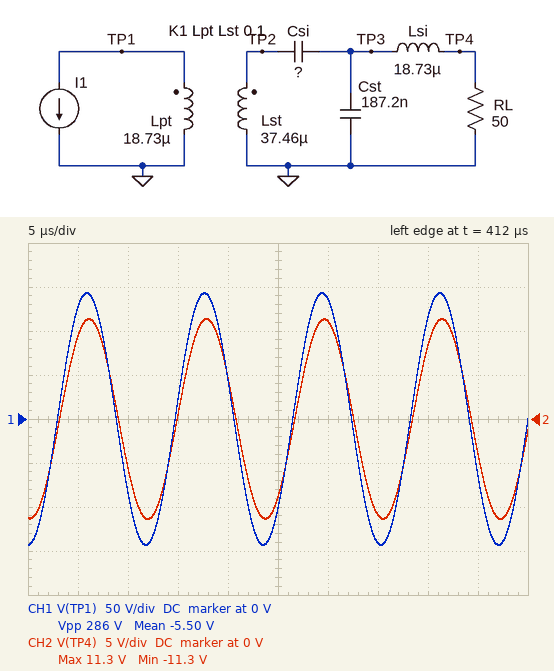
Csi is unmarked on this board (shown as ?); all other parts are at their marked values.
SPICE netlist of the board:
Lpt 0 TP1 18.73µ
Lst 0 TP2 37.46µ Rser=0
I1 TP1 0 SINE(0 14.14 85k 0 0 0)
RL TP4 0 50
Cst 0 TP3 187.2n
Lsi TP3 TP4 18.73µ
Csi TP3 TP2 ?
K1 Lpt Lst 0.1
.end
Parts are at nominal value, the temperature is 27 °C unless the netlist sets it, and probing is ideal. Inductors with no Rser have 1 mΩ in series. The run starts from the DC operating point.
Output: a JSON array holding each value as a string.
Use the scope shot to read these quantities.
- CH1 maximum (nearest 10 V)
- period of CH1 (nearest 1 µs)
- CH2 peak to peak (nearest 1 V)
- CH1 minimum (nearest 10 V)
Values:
["140 V", "12 µs", "23 V", "-140 V"]
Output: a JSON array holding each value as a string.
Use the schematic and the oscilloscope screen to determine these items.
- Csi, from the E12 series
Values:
["68 nF"]
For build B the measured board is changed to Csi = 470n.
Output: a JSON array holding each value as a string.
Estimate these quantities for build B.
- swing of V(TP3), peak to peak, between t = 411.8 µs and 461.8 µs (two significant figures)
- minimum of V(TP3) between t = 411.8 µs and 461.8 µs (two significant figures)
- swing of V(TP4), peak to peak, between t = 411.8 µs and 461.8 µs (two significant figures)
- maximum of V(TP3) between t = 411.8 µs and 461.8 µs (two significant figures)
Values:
["64 V", "-32 V", "63 V", "32 V"]
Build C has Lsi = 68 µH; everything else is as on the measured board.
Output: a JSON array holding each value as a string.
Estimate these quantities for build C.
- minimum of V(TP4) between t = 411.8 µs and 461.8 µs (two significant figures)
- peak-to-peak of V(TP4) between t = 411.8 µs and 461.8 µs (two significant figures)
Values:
["-9.9 V", "20 V"]
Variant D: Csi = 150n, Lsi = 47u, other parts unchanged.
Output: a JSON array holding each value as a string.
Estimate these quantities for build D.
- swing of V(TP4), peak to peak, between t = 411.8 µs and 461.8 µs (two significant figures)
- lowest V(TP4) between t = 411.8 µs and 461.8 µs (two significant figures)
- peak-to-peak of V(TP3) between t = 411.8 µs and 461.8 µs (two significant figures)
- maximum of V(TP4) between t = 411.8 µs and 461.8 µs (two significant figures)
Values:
["110 V", "-54 V", "120 V", "54 V"]
